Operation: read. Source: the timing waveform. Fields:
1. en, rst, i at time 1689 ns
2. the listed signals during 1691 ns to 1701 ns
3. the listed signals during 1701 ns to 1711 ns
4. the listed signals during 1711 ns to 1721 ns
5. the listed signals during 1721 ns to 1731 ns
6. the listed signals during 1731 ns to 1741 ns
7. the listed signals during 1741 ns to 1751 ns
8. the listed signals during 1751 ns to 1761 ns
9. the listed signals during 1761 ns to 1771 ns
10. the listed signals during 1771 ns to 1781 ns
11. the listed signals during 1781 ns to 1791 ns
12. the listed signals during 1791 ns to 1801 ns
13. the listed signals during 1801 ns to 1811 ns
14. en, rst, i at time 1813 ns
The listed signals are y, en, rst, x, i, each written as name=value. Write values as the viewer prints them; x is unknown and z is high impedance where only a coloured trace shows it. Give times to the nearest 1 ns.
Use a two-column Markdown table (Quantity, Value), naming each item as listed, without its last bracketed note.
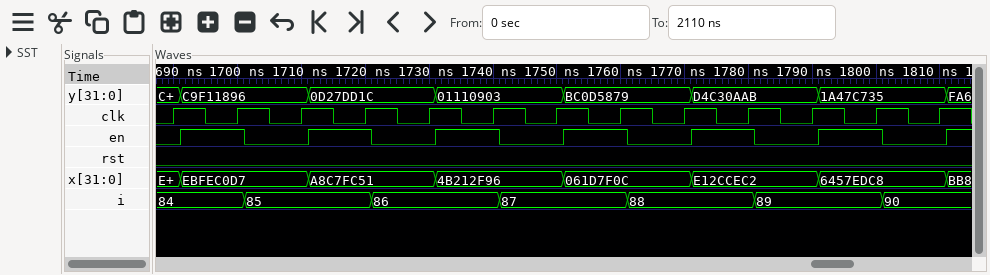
| Quantity | Value |
|---|---|
| en, rst, i at time 1689 ns | en=0, rst=0, i=84 |
| the listed signals during 1691 ns to 1701 ns | y=C9F11896, en=1, rst=0, x=EBFEC0D7, i=84 |
| the listed signals during 1701 ns to 1711 ns | y=C9F11896, en=0, rst=0, x=EBFEC0D7, i=85 |
| the listed signals during 1711 ns to 1721 ns | y=0D27DD1C, en=1, rst=0, x=A8C7FC51, i=85 |
| the listed signals during 1721 ns to 1731 ns | y=0D27DD1C, en=0, rst=0, x=A8C7FC51, i=86 |
| the listed signals during 1731 ns to 1741 ns | y=01110903, en=1, rst=0, x=4B212F96, i=86 |
| the listed signals during 1741 ns to 1751 ns | y=01110903, en=0, rst=0, x=4B212F96, i=87 |
| the listed signals during 1751 ns to 1761 ns | y=BC0D5879, en=1, rst=0, x=061D7F0C, i=87 |
| the listed signals during 1761 ns to 1771 ns | y=BC0D5879, en=0, rst=0, x=061D7F0C, i=88 |
| the listed signals during 1771 ns to 1781 ns | y=D4C30AAB, en=1, rst=0, x=E12CCEC2, i=88 |
| the listed signals during 1781 ns to 1791 ns | y=D4C30AAB, en=0, rst=0, x=E12CCEC2, i=89 |
| the listed signals during 1791 ns to 1801 ns | y=1A47C735, en=1, rst=0, x=6457EDC8, i=89 |
| the listed signals during 1801 ns to 1811 ns | y=1A47C735, en=0, rst=0, x=6457EDC8, i=90 |
| en, rst, i at time 1813 ns | en=1, rst=0, i=90 |
